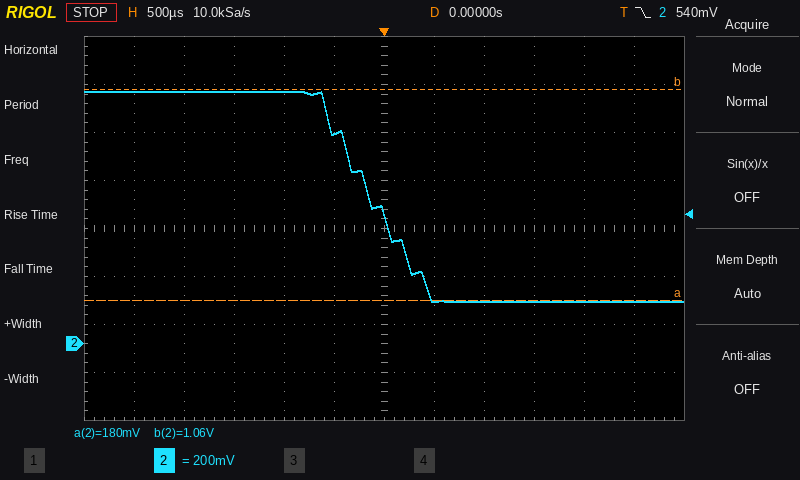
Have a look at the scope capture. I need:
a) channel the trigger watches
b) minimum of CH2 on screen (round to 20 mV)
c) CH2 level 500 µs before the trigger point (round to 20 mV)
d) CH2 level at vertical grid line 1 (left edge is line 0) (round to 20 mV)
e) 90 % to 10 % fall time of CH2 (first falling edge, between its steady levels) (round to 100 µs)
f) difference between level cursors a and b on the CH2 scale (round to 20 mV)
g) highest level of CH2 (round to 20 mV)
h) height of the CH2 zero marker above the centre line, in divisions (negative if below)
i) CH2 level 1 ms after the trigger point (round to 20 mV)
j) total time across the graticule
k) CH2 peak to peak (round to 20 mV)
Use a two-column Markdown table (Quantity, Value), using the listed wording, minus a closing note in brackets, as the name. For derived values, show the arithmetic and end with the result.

| Quantity | Value |
|---|---|
| channel the trigger watches | CH2 |
| minimum of CH2 on screen | 180 mV |
| CH2 level 500 µs before the trigger point | 880 mV |
| CH2 level at vertical grid line 1 (left edge is line 0) | 1.06 V |
| 90 % to 10 % fall time of CH2 (first falling edge, between its steady levels) | 1.0 ms |
| difference between level cursors a and b on the CH2 scale | 880 mV |
| highest level of CH2 | 1.06 V |
| height of the CH2 zero marker above the centre line, in divisions | -2.4 div |
| CH2 level 1 ms after the trigger point | 180 mV |
| total time across the graticule | 6 ms |
| CH2 peak to peak | 1.06 V − (180 mV) = 880 mV |
